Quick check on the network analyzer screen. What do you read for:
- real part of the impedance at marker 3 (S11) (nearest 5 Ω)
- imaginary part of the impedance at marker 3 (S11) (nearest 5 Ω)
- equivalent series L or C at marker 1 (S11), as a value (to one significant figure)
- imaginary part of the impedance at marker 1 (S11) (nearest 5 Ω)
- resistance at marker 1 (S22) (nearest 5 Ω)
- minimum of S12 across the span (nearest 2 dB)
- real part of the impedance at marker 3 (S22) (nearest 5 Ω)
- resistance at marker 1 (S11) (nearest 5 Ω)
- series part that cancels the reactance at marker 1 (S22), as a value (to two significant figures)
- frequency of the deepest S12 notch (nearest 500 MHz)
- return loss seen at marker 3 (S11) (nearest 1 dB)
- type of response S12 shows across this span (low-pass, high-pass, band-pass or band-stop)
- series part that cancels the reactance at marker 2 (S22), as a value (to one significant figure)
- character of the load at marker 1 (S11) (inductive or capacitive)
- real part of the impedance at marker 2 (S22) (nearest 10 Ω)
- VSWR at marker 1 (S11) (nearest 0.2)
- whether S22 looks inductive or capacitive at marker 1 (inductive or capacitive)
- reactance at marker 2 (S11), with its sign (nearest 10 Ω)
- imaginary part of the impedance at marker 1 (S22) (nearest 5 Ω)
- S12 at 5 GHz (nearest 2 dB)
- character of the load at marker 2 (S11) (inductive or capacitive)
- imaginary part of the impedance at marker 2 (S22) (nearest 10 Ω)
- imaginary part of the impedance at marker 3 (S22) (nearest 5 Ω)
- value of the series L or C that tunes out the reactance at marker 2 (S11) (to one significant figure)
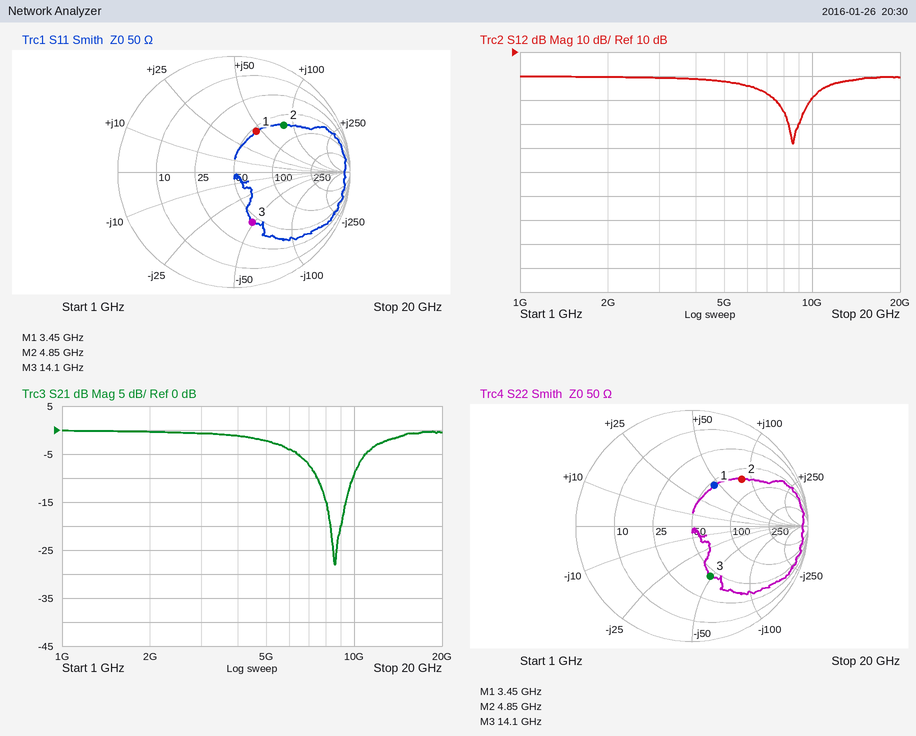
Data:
45 Ω
-50 Ω
2 nH
+45 Ω
55 Ω
-28 dB
45 Ω
55 Ω
1.0 pF
8.5 GHz
7 dB
band-stop
400 fF
inductive
70 Ω
2.4
inductive
+80 Ω
+45 Ω
-2 dB
inductive
+80 Ω
-50 Ω
400 fF
